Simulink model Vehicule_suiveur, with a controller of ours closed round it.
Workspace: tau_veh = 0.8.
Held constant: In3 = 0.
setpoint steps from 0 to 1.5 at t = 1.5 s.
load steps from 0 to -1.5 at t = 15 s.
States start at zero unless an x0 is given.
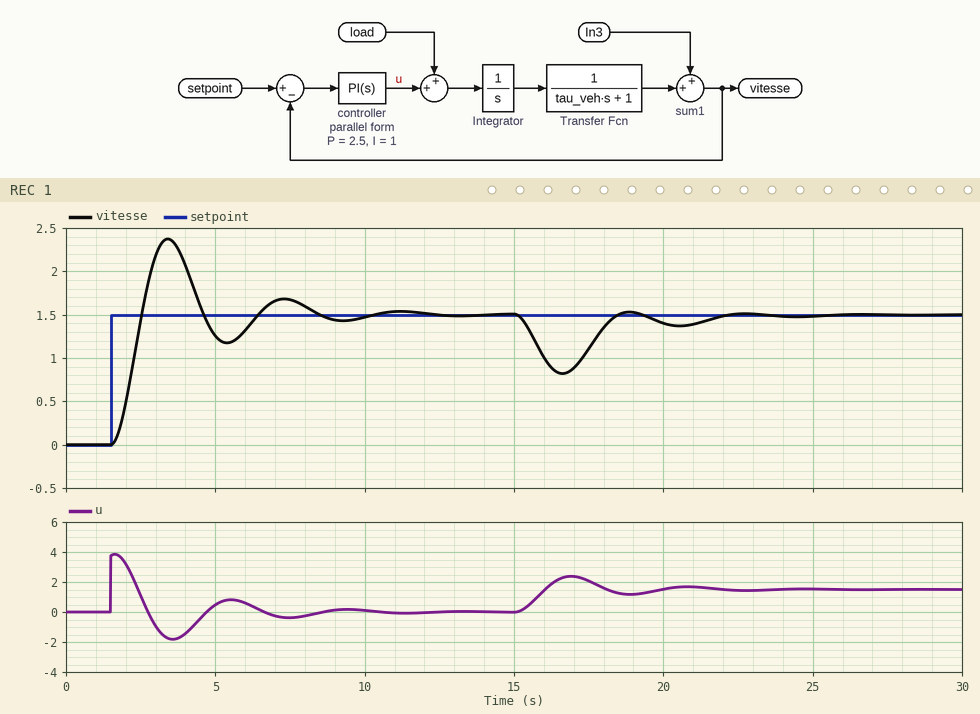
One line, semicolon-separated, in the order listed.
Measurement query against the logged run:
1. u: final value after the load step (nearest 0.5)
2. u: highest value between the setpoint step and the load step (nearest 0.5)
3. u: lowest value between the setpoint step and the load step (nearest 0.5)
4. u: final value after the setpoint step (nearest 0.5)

1.5; 4.0; -2.0; 0.0
